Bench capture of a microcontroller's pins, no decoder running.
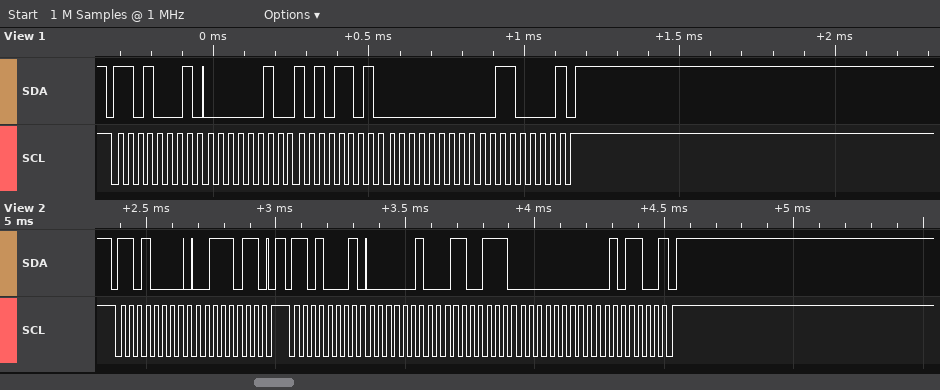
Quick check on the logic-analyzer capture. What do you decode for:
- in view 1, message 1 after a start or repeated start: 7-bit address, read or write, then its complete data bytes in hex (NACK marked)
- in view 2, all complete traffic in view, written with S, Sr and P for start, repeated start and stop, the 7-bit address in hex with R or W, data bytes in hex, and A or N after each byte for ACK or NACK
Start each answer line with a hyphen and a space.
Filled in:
- 0x68 read: 02 AD 00 30 NACK
- S 68W A 3B A P S 68R A 02 A 67 A 00 A 2C N P
